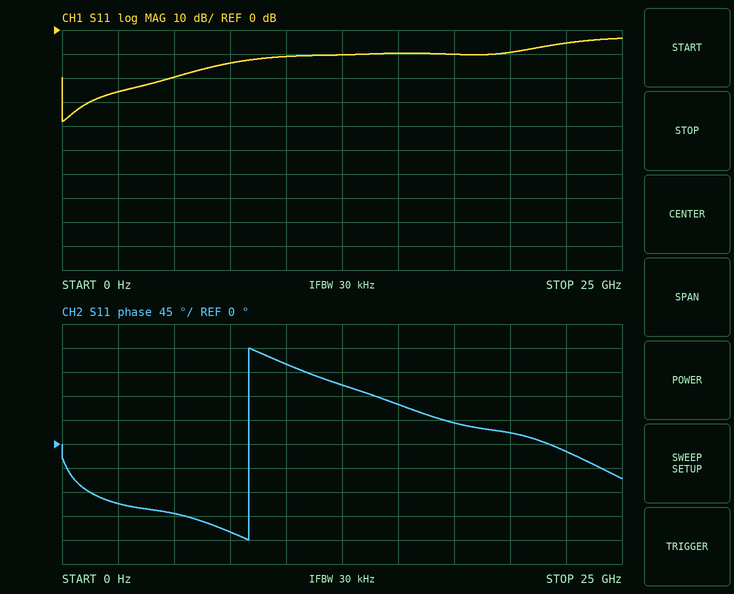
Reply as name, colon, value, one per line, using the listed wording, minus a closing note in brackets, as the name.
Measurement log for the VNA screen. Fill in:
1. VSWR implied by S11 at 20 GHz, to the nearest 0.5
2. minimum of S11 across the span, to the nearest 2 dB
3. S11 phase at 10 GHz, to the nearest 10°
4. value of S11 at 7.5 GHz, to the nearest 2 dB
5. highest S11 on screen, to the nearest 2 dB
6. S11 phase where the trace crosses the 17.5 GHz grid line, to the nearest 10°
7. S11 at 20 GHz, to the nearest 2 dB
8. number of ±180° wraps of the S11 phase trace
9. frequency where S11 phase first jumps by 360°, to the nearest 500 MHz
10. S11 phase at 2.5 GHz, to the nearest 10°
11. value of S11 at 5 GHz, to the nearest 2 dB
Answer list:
VSWR implied by S11 at 20 GHz, to the nearest 0.5: 2.0
minimum of S11 across the span, to the nearest 2 dB: -38 dB
S11 phase at 10 GHz, to the nearest 10°: 150°
value of S11 at 7.5 GHz, to the nearest 2 dB: -14 dB
highest S11 on screen, to the nearest 2 dB: -4 dB
S11 phase where the trace crosses the 17.5 GHz grid line, to the nearest 10°: 40°
S11 at 20 GHz, to the nearest 2 dB: -10 dB
number of ±180° wraps of the S11 phase trace: 1
frequency where S11 phase first jumps by 360°, to the nearest 500 MHz: 8.5 GHz
S11 phase at 2.5 GHz, to the nearest 10°: -110°
value of S11 at 5 GHz, to the nearest 2 dB: -20 dB
